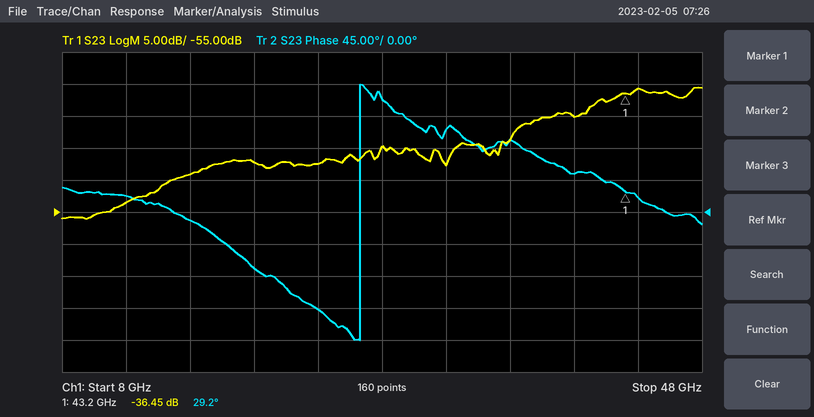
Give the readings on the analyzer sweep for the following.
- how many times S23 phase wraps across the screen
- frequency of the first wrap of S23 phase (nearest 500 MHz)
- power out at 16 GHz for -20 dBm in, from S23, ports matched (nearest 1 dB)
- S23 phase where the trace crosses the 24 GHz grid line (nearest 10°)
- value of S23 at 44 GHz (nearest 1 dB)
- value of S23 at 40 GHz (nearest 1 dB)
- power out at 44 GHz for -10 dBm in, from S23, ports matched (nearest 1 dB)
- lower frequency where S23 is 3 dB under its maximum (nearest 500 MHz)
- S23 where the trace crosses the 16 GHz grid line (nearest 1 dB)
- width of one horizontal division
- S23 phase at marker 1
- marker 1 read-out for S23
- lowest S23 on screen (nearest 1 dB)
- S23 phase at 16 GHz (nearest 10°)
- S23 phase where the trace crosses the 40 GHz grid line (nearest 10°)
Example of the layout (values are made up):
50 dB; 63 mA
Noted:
1; 26.5 GHz; -69 dBm; -140°; -36 dB; -40 dB; -46 dBm; 41.0 GHz; -49 dB; 4 GHz; 29.2°; -36.45 dB; -56 dB; -10°; 50°
